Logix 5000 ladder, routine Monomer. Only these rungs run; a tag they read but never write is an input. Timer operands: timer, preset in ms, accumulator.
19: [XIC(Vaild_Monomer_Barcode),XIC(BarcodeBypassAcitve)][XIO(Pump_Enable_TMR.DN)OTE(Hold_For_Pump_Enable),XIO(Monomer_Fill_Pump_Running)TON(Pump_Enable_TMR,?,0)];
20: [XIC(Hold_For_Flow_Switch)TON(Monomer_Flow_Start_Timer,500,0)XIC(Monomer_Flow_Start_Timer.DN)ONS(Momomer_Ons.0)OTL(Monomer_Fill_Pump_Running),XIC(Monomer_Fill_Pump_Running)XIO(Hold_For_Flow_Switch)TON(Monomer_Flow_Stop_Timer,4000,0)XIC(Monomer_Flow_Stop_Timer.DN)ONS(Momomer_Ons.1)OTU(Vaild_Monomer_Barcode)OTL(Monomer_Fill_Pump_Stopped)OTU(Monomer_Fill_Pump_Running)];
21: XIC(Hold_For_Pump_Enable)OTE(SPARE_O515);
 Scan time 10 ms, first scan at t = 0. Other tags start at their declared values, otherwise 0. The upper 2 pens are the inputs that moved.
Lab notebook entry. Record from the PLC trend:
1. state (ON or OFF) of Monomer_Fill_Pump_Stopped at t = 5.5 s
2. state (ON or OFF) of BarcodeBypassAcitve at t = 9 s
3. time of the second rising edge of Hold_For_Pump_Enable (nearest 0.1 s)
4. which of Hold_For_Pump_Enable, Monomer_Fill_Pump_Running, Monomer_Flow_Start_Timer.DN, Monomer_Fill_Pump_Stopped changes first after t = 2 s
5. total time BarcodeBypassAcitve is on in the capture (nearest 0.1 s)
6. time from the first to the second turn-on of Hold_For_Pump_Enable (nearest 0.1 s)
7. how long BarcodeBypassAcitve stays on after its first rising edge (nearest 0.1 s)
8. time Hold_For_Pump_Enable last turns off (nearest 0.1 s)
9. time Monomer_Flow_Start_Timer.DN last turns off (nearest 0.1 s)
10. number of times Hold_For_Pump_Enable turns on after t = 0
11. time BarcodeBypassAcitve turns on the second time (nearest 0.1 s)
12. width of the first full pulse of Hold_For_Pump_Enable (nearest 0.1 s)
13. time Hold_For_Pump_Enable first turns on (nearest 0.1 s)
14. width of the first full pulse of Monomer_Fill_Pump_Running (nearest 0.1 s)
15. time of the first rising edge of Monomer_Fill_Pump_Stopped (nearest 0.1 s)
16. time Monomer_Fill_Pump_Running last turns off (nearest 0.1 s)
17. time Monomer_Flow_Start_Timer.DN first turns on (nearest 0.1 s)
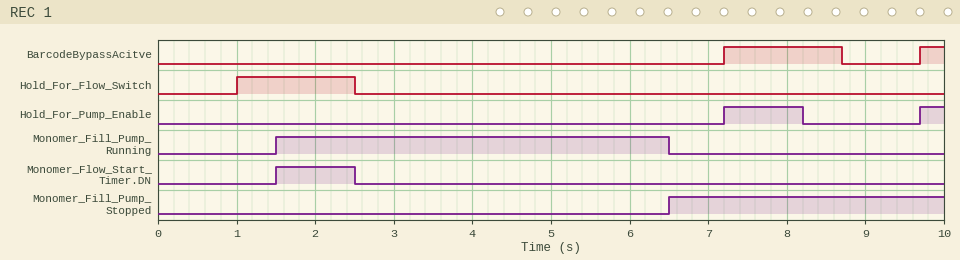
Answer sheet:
OFF
OFF
9.7 s
Monomer_Flow_Start_Timer.DN
1.8 s
2.5 s
1.5 s
8.2 s
2.5 s
2
9.7 s
1.0 s
7.2 s
5.0 s
6.5 s
6.5 s
1.5 s
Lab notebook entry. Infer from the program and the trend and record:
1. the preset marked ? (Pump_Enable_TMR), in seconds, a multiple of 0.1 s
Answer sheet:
1.0 s
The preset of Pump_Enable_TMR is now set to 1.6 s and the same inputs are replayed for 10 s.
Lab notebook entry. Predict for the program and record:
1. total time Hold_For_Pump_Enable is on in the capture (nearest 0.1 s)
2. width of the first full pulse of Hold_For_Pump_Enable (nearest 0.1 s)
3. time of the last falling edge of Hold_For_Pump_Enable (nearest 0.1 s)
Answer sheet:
1.8 s
1.5 s
8.7 s
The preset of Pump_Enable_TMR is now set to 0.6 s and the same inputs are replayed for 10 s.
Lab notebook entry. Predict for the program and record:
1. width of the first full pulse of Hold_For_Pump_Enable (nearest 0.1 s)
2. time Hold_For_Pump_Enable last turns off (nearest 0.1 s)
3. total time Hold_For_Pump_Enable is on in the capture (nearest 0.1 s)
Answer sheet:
0.6 s
7.8 s
0.9 s
